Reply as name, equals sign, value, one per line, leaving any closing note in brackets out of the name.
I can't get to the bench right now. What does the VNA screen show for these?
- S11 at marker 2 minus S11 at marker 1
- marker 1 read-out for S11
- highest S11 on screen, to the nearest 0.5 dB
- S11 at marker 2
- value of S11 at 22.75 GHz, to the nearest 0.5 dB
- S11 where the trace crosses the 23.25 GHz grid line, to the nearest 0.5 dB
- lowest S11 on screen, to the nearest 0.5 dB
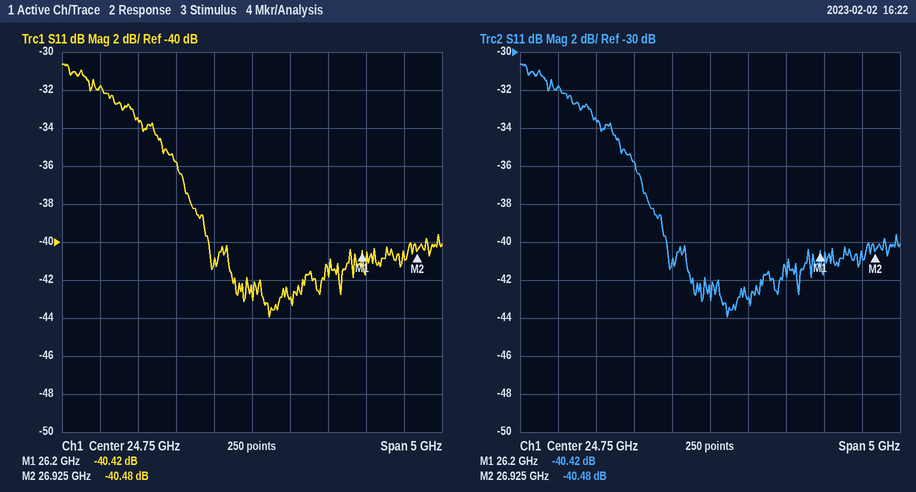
S11 at marker 2 minus S11 at marker 1 = -0.06 dB
marker 1 read-out for S11 = -40.42 dB
highest S11 on screen, to the nearest 0.5 dB = -30.5 dB
S11 at marker 2 = -40.48 dB
value of S11 at 22.75 GHz, to the nearest 0.5 dB = -32.0 dB
S11 where the trace crosses the 23.25 GHz grid line, to the nearest 0.5 dB = -33.5 dB
lowest S11 on screen, to the nearest 0.5 dB = -44.0 dB
